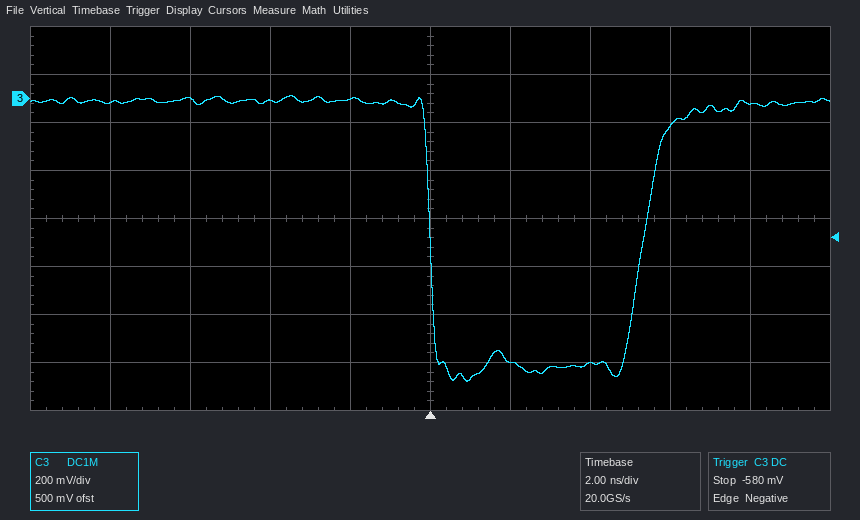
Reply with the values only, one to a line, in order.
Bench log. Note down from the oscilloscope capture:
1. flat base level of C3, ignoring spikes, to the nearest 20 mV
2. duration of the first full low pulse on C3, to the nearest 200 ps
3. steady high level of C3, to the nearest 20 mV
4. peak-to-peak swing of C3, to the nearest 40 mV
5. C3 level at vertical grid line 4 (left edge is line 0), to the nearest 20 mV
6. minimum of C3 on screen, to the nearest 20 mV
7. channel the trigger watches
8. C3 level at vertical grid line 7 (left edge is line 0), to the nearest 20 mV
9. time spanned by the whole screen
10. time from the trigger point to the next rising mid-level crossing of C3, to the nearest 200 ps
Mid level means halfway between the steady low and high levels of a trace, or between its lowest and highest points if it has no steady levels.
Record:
-1.12 V
5.4 ns
-20 mV
1.20 V
0 mV
-1.18 V
C3
-1.10 V
20 ns
5.4 ns
